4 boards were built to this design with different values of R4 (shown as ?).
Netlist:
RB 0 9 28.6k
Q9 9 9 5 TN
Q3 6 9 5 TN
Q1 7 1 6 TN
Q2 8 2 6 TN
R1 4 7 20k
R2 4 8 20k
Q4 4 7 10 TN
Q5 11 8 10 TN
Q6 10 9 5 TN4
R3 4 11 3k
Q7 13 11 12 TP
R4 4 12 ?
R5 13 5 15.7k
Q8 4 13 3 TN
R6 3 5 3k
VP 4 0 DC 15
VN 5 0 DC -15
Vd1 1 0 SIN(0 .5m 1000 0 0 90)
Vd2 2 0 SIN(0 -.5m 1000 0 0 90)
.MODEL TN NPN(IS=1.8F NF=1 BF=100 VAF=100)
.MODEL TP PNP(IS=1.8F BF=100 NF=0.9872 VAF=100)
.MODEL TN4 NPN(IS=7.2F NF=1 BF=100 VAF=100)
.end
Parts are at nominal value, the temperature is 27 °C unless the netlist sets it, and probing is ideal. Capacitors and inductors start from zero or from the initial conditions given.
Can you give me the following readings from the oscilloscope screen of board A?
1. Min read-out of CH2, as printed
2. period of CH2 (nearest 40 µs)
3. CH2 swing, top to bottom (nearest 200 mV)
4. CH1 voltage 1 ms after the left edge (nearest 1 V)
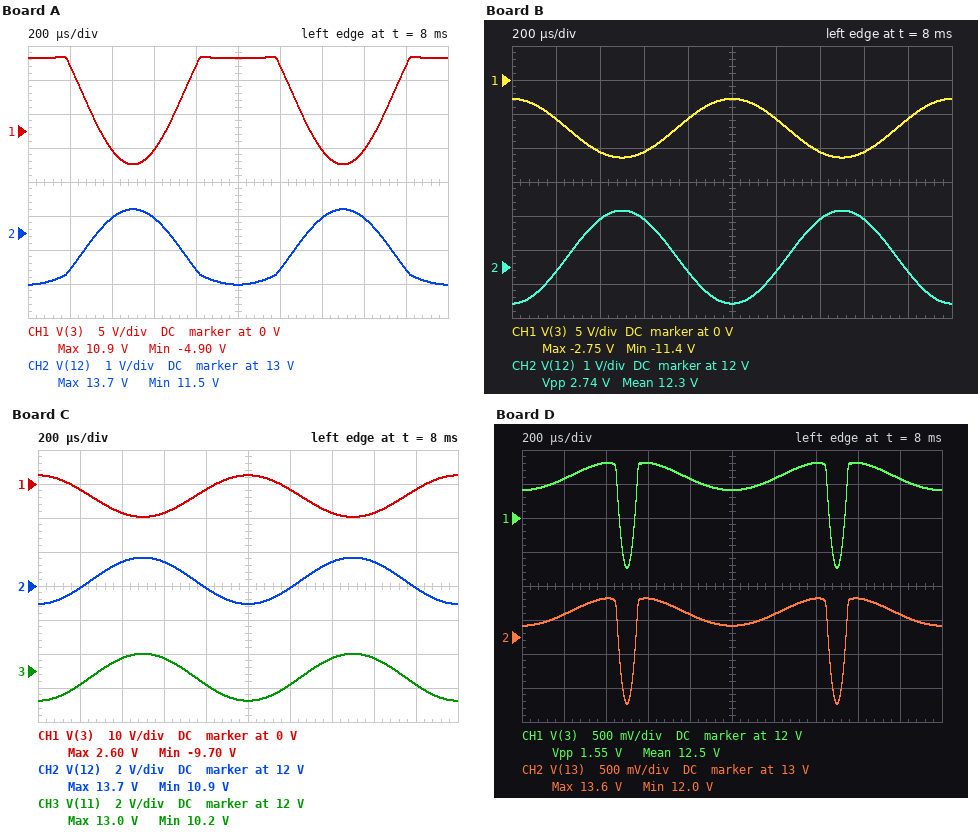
11.5 V
1.00 ms
2.2 V
11 V
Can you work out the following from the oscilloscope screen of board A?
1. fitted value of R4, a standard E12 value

1.8 kΩ
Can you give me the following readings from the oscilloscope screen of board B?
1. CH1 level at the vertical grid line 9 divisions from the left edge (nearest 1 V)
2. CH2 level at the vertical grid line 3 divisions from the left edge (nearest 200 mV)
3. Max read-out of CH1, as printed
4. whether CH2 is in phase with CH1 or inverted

-6 V
13.4 V
-2.75 V
inverted
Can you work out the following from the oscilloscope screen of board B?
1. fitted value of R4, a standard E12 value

4.7 kΩ
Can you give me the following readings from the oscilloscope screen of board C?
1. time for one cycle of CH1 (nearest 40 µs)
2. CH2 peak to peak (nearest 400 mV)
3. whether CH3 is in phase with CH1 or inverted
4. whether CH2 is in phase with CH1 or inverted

1.00 ms
2.8 V
inverted
inverted
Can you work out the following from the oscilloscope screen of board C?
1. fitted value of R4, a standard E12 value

3.3 kΩ
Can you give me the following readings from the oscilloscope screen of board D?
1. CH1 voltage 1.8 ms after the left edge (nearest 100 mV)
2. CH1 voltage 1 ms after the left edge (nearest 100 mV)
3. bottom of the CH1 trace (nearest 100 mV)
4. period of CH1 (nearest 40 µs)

12.6 V
12.4 V
11.3 V
1.00 ms
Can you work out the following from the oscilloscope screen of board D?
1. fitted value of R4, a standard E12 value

680 Ω
